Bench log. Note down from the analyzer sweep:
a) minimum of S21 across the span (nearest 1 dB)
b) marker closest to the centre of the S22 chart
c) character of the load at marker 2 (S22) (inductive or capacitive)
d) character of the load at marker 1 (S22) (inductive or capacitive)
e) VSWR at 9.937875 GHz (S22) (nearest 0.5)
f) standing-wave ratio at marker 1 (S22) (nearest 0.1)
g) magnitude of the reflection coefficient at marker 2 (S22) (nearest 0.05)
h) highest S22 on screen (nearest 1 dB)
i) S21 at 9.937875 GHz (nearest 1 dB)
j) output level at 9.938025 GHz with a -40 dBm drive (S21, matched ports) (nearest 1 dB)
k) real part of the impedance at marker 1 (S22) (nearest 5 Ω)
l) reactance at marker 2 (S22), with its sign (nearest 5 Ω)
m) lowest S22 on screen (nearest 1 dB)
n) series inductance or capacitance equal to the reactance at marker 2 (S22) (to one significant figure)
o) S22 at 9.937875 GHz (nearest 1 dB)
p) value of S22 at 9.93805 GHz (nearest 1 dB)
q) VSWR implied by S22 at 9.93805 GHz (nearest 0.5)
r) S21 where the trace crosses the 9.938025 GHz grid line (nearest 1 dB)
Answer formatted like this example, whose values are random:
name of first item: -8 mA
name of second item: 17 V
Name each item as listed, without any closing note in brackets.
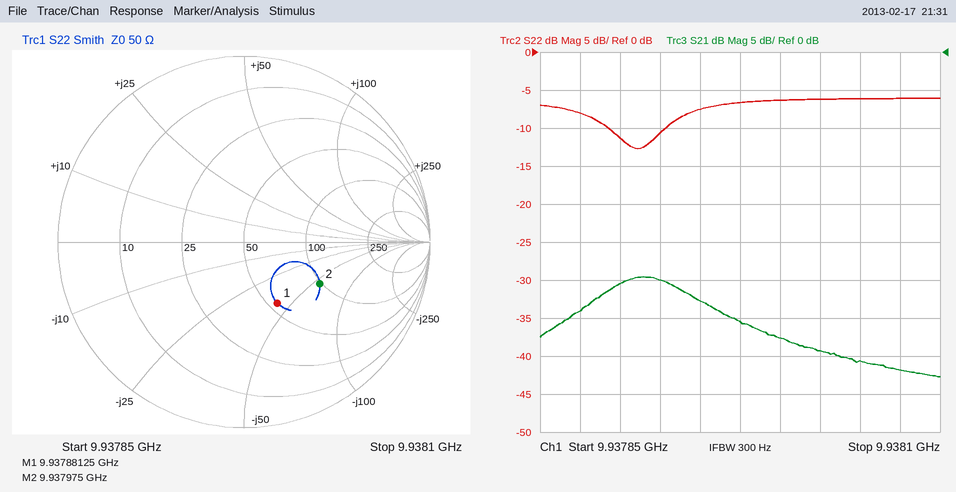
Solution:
minimum of S21 across the span: -43 dB
marker closest to the centre of the S22 chart: marker 1
character of the load at marker 2 (S22): capacitive
character of the load at marker 1 (S22): capacitive
VSWR at 9.937875 GHz (S22): 2.5
standing-wave ratio at marker 1 (S22): 2.2
magnitude of the reflection coefficient at marker 2 (S22): 0.45
highest S22 on screen: -6 dB
S21 at 9.937875 GHz: -34 dB
output level at 9.938025 GHz with a -40 dBm drive (S21, matched ports): -79 dBm
real part of the impedance at marker 1 (S22): 55 Ω
reactance at marker 2 (S22), with its sign: -55 Ω
lowest S22 on screen: -13 dB
series inductance or capacitance equal to the reactance at marker 2 (S22): 300 fF
S22 at 9.937875 GHz: -8 dB
value of S22 at 9.93805 GHz: -6 dB
VSWR implied by S22 at 9.93805 GHz: 3.0
S21 where the trace crosses the 9.938025 GHz grid line: -39 dB
